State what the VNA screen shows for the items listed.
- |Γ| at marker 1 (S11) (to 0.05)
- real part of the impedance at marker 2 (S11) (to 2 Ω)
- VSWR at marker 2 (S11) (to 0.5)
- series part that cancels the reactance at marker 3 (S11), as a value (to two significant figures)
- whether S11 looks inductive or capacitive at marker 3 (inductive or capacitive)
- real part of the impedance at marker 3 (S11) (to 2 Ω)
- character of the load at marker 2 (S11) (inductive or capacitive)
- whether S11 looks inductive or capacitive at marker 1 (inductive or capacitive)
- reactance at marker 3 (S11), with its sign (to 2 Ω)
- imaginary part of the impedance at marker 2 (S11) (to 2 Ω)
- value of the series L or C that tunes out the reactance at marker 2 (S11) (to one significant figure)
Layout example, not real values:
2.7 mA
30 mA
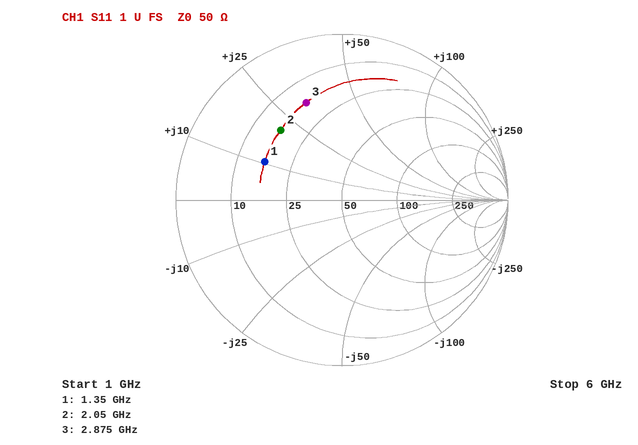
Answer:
0.50
16 Ω
3.5
1.7 pF
inductive
16 Ω
inductive
inductive
+32 Ω
+20 Ω
4 pF
